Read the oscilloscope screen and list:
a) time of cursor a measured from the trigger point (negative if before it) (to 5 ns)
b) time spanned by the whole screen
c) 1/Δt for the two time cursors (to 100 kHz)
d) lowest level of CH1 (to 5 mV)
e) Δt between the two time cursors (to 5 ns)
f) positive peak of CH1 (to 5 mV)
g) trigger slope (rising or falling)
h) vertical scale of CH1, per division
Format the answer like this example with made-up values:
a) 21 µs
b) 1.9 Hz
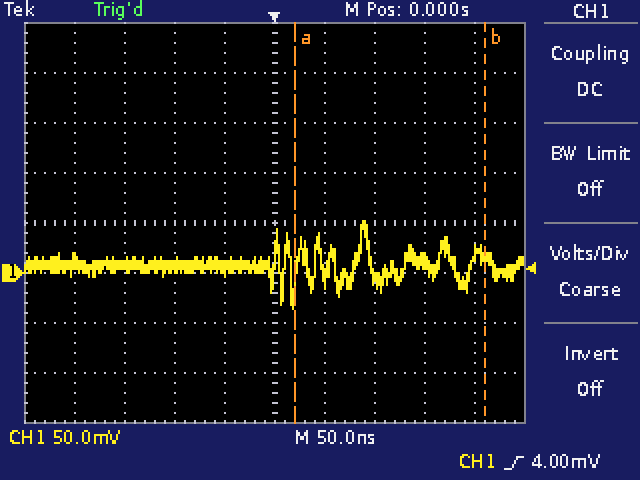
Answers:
a) +20 ns
b) 500 ns
c) 5.3 MHz
d) -35 mV
e) 190 ns
f) 50 mV
g) rising
h) 50 mV
